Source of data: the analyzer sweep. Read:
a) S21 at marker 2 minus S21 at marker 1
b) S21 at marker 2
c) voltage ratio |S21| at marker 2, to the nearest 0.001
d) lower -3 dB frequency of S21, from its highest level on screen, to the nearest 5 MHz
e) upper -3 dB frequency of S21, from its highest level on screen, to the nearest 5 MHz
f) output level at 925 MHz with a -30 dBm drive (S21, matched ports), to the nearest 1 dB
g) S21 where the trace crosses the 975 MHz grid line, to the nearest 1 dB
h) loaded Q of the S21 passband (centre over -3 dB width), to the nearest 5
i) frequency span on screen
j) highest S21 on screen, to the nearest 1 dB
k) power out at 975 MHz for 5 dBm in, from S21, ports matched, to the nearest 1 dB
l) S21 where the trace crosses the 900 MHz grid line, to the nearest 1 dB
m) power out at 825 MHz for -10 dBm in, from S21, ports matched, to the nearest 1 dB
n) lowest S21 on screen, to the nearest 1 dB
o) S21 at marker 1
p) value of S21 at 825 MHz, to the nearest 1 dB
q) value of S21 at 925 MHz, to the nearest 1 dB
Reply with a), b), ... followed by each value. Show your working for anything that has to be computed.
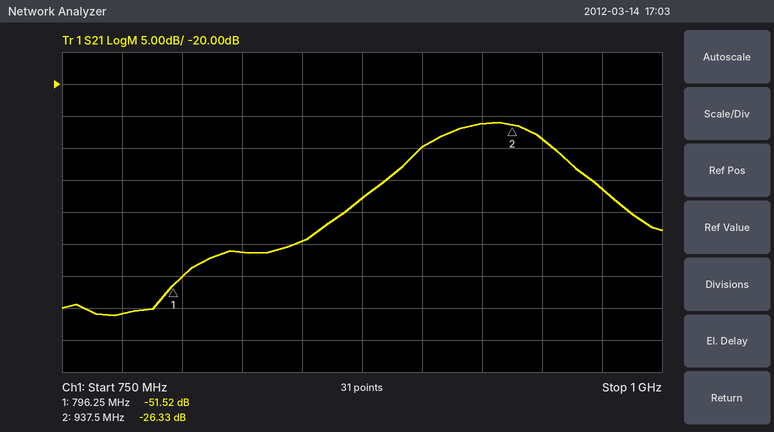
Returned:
a) -26.33 − (-51.52) = 25.19 dB
b) -26.33 dB
c) 10^(-26.33/20) ≈ 0.048
d) 905 MHz
e) 950 MHz
f) -30 dBm + (-26 dB) = -56 dBm
g) -36 dB
h) 927.5 MHz / 45 MHz ≈ 20.6, so 20 to the nearest 5
i) 250 MHz
j) -26 dB
k) 5 dBm + (-36 dB) = -31 dBm
l) -30 dB
m) -10 dBm + (-46 dB) = -56 dBm
n) -56 dB
o) -51.52 dB
p) -46 dB
q) -26 dB
